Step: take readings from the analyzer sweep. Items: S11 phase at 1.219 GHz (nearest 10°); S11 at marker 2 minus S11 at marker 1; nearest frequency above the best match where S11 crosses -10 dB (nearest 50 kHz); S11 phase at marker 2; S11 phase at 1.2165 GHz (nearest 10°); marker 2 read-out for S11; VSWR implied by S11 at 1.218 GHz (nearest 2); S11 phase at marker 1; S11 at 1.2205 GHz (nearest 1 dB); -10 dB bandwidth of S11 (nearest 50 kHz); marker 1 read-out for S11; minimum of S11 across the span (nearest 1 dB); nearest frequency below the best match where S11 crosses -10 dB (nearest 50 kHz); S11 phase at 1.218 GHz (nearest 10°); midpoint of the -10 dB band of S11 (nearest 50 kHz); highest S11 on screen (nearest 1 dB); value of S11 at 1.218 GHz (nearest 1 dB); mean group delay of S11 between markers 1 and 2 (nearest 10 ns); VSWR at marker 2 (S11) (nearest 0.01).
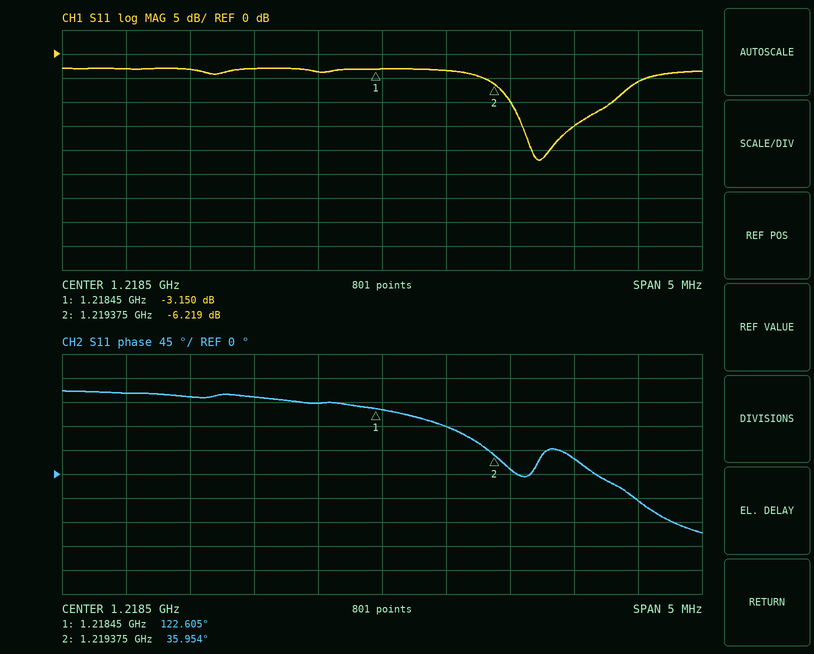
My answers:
90°
-3.069 dB
1.22030 GHz
35.954°
150°
-6.219 dB
4
122.605°
-6 dB
800 kHz
-3.150 dB
-22 dB
1.21950 GHz
130°
1.21990 GHz
-3 dB
-4 dB
260 ns
2.91
